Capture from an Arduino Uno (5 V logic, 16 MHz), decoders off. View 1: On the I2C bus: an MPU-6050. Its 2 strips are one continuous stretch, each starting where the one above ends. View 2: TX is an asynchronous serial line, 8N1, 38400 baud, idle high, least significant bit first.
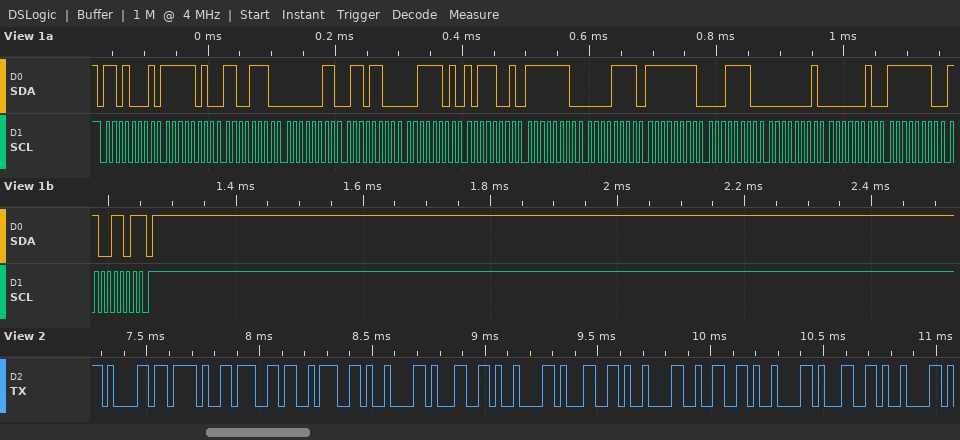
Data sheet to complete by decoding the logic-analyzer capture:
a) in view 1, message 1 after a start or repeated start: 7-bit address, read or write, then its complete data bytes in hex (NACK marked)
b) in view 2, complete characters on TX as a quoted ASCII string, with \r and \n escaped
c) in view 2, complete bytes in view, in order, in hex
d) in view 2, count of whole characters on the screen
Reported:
0x68 read: FA CE 03 6C 3D B9 FE 0F FF 1E 01 02 FE CD NACK
"a/g:\t1\t1\t2\t1\t"
61 2F 67 3A 09 31 09 31 09 32 09 31 09
13
